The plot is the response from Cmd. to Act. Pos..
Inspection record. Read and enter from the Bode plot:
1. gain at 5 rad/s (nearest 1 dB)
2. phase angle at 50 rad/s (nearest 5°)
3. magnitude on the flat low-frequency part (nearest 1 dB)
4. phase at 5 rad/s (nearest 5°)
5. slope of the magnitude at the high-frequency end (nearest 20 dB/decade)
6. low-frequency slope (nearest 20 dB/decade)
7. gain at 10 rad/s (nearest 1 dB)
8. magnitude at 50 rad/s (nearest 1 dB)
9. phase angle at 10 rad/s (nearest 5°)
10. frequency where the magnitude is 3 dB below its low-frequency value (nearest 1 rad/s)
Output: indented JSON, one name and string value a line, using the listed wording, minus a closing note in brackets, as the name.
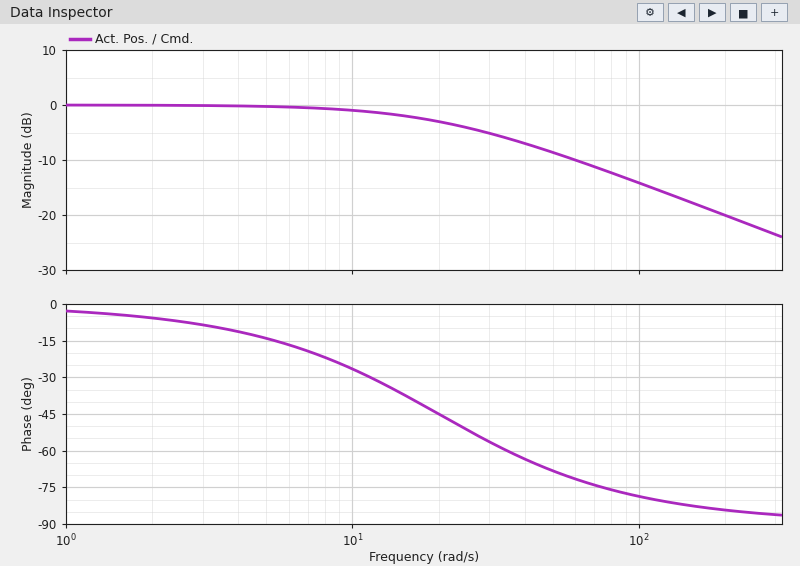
{
  "gain at 5 rad/s": "0 dB",
  "phase angle at 50 rad/s": "-70°",
  "magnitude on the flat low-frequency part": "0 dB",
  "phase at 5 rad/s": "-15°",
  "slope of the magnitude at the high-frequency end": "-20 dB/decade",
  "low-frequency slope": "0 dB/decade",
  "gain at 10 rad/s": "-1 dB",
  "magnitude at 50 rad/s": "-9 dB",
  "phase angle at 10 rad/s": "-25°",
  "frequency where the magnitude is 3 dB below its low-frequency value": "20 rad/s"
}
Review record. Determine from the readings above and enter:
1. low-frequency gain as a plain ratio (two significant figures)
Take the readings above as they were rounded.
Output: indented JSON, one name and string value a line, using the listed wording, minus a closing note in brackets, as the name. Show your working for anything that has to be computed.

{
  "low-frequency gain as a plain ratio": "10^(0 / 20) = 1.0"
}
